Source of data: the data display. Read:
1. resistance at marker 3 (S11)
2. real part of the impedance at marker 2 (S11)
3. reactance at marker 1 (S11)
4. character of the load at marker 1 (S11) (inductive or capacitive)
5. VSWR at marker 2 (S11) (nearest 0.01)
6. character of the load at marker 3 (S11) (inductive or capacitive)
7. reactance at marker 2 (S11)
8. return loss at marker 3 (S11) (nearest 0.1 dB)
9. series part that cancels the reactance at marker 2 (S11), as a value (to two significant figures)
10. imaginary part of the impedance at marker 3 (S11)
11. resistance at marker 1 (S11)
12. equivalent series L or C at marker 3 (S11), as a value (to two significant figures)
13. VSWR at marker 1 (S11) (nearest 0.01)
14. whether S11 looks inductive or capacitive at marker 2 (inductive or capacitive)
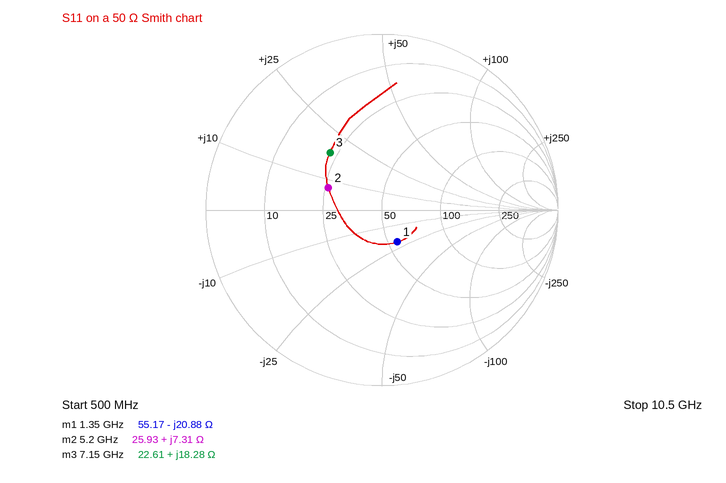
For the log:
22.61 Ω
25.93 Ω
-20.88 Ω
capacitive
1.98
inductive
+7.31 Ω
7.1 dB
4.2 pF
+18.28 Ω
55.17 Ω
410 pH
1.50
inductive
